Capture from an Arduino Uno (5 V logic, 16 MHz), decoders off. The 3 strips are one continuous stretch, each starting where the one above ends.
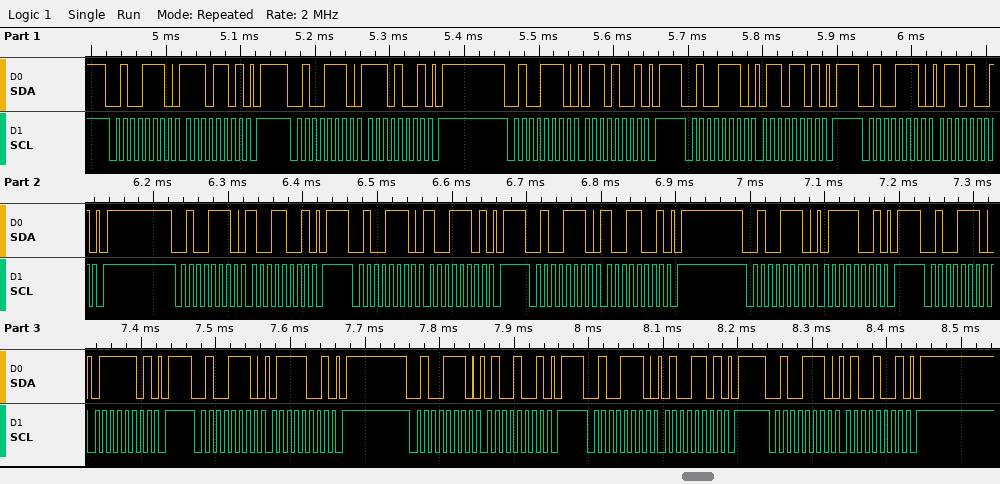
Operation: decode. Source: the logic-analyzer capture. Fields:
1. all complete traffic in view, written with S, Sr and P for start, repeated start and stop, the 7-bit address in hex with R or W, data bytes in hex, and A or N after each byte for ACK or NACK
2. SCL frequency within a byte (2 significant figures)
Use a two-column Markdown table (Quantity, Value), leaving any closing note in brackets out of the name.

| Quantity | Value |
|---|---|
| all complete traffic in view, written with S, Sr and P for start, repeated start and stop, the 7-bit address in hex with R or W, data bytes in hex, and A or N after each byte for ACK or NACK | S 27W A ED A P S 27W A E9 A P S 27W A 69 A P S 27W A 6D A P S 27W A 69 A P S 27W A 99 A P S 27W A 9D A P S 27W A 99 A P S 27W A 79 A P S 27W A 7D A P S 27W A 79 A P S 27W A 49 A P S 27W A 4D A P S 27W A 49 A P |
| SCL frequency within a byte | 100 kHz |
